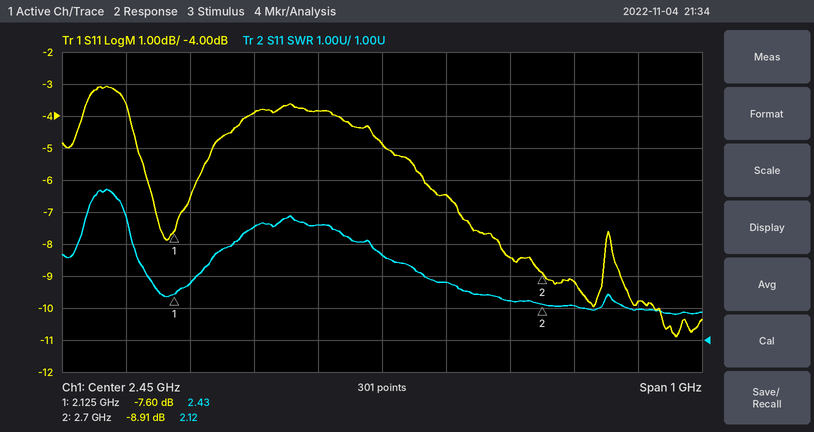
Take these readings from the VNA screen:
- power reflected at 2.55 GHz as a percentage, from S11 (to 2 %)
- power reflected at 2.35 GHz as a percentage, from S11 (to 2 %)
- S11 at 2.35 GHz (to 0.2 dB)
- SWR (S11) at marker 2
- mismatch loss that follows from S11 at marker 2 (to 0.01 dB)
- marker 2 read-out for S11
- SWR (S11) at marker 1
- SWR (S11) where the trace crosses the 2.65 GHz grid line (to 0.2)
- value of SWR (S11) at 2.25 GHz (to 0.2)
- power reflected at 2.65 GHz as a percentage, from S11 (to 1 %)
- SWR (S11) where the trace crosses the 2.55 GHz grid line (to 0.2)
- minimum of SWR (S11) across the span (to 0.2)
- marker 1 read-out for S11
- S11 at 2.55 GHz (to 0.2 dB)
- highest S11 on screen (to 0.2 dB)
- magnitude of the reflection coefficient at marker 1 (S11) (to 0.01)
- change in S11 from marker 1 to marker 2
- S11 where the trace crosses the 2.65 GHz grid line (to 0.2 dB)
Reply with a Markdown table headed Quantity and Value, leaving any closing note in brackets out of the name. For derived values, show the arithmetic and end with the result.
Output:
| Quantity | Value |
|---|---|
| power reflected at 2.55 GHz as a percentage, from S11 | 10^(-6.4/10) ≈ 22.9 %, so 22 % to the nearest 2 % |
| power reflected at 2.35 GHz as a percentage, from S11 | 10^(-3.8/10) ≈ 42 % |
| S11 at 2.35 GHz | -3.8 dB |
| SWR (S11) at marker 2 | 2.12 |
| mismatch loss that follows from S11 at marker 2 | −10 log10(1 − 10^(-8.91/10)) ≈ 0.60 dB |
| marker 2 read-out for S11 | -8.91 dB |
| SWR (S11) at marker 1 | 2.43 |
| SWR (S11) where the trace crosses the 2.65 GHz grid line | 2.2 |
| value of SWR (S11) at 2.25 GHz | 4.6 |
| power reflected at 2.65 GHz as a percentage, from S11 | 10^(-8.4/10) ≈ 14 % |
| SWR (S11) where the trace crosses the 2.55 GHz grid line | 2.8 |
| minimum of SWR (S11) across the span | 1.8 |
| marker 1 read-out for S11 | -7.60 dB |
| S11 at 2.55 GHz | -6.4 dB |
| highest S11 on screen | -3.0 dB |
| magnitude of the reflection coefficient at marker 1 (S11) | 10^(-7.6/20) ≈ 0.42 |
| change in S11 from marker 1 to marker 2 | -8.91 − (-7.6) = -1.31 dB |
| S11 where the trace crosses the 2.65 GHz grid line | -8.4 dB |
